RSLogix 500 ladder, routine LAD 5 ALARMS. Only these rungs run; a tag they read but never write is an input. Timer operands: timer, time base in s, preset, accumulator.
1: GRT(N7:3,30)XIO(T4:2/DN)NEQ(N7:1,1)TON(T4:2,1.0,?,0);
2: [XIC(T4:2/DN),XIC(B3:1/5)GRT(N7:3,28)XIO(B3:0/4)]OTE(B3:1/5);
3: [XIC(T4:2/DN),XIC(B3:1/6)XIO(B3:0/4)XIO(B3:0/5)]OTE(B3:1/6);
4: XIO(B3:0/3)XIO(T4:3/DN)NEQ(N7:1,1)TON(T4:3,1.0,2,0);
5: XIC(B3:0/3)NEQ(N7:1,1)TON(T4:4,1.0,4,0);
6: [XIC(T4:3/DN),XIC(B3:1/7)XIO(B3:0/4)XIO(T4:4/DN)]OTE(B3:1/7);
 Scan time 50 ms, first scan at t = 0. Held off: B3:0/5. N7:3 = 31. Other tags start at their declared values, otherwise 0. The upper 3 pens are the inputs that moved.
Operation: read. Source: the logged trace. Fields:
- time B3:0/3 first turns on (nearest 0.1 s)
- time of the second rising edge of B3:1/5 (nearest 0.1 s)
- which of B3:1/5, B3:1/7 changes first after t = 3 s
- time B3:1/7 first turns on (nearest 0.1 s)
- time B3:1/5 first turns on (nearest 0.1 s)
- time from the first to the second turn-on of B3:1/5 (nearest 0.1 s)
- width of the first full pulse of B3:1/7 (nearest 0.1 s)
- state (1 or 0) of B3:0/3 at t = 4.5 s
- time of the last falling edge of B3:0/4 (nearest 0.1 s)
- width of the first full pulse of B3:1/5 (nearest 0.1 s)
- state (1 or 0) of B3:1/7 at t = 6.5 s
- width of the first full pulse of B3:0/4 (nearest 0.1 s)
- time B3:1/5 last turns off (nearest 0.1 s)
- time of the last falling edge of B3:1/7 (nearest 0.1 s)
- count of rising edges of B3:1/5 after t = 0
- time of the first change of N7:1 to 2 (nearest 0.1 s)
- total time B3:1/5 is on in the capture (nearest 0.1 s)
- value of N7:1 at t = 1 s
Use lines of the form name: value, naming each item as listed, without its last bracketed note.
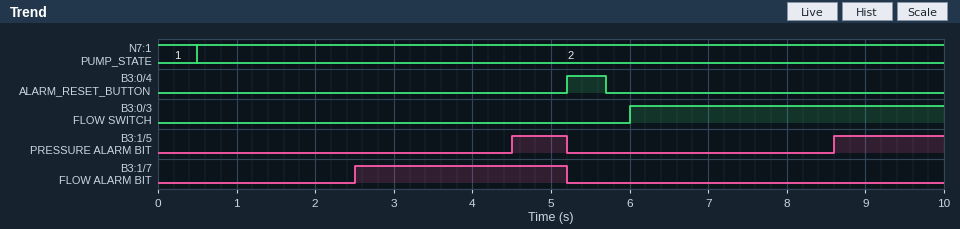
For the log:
time B3:0/3 first turns on: 6.0 s
time of the second rising edge of B3:1/5: 8.6 s
which of B3:1/5, B3:1/7 changes first after t = 3 s: B3:1/5
time B3:1/7 first turns on: 2.5 s
time B3:1/5 first turns on: 4.5 s
time from the first to the second turn-on of B3:1/5: 4.1 s
width of the first full pulse of B3:1/7: 2.7 s
state (1 or 0) of B3:0/3 at t = 4.5 s: 0
time of the last falling edge of B3:0/4: 5.7 s
width of the first full pulse of B3:1/5: 0.7 s
state (1 or 0) of B3:1/7 at t = 6.5 s: 0
width of the first full pulse of B3:0/4: 0.5 s
time B3:1/5 last turns off: 5.2 s
time of the last falling edge of B3:1/7: 5.2 s
count of rising edges of B3:1/5 after t = 0: 2
time of the first change of N7:1 to 2: 0.5 s
total time B3:1/5 is on in the capture: 2.1 s
value of N7:1 at t = 1 s: 2
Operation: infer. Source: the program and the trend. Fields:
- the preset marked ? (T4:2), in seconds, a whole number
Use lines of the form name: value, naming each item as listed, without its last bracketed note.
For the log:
the preset marked ? (T4:2), in seconds, a whole number: 4 s
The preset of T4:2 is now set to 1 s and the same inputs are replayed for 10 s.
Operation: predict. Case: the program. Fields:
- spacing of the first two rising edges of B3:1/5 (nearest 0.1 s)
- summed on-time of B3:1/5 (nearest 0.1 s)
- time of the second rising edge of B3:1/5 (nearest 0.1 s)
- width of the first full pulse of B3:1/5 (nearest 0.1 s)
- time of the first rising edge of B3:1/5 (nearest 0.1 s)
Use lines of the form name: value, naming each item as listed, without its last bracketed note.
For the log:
spacing of the first two rising edges of B3:1/5: 4.4 s
summed on-time of B3:1/5: 7.8 s
time of the second rising edge of B3:1/5: 5.9 s
width of the first full pulse of B3:1/5: 3.7 s
time of the first rising edge of B3:1/5: 1.5 s
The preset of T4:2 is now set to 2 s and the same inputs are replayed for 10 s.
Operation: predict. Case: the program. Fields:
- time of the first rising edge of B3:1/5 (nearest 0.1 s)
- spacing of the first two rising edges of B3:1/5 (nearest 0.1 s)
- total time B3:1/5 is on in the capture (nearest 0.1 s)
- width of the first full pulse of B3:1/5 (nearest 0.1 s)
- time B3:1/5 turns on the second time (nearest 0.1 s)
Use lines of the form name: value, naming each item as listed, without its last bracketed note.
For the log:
time of the first rising edge of B3:1/5: 2.5 s
spacing of the first two rising edges of B3:1/5: 4.2 s
total time B3:1/5 is on in the capture: 6.0 s
width of the first full pulse of B3:1/5: 2.7 s
time B3:1/5 turns on the second time: 6.7 s
